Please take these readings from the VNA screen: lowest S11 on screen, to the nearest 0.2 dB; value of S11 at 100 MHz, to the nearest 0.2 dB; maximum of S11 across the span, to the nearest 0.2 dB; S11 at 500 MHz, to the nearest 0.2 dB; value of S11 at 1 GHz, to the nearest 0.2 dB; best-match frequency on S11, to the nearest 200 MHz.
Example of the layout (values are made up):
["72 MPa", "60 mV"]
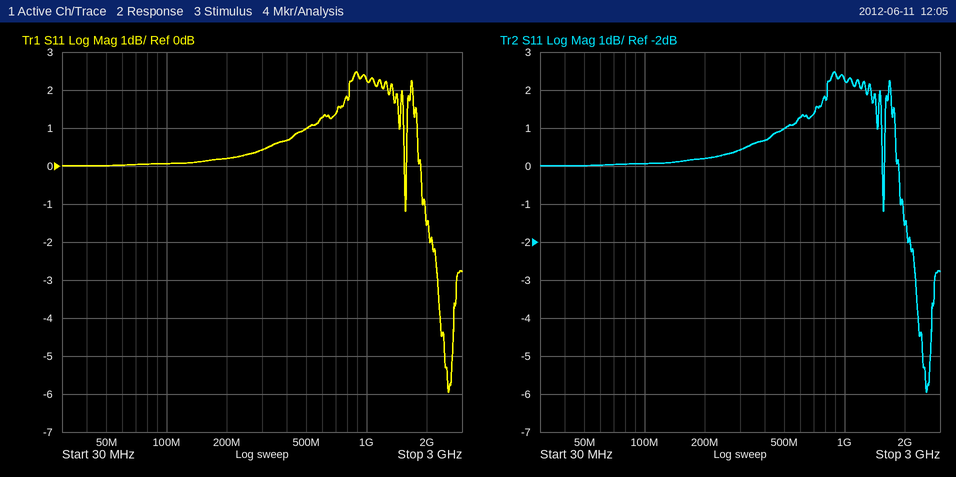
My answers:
["-6.0 dB", "0.0 dB", "2.4 dB", "1.0 dB", "2.2 dB", "2.6 GHz"]
